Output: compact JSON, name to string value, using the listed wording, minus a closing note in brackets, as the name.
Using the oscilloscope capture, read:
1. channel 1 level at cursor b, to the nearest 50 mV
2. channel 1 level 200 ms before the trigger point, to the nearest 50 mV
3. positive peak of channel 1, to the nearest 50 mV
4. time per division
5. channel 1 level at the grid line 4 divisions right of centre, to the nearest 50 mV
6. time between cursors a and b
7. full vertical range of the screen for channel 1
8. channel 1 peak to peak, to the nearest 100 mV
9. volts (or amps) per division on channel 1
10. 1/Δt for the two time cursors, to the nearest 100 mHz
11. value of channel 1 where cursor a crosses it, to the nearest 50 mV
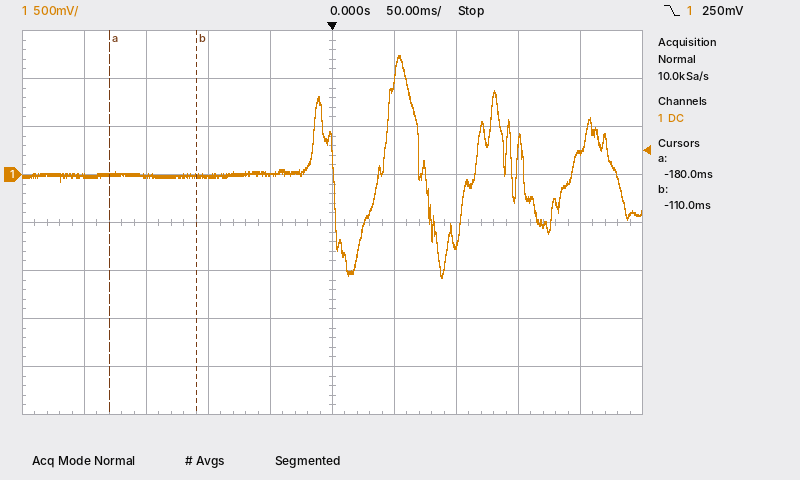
{"channel 1 level at cursor b, to the nearest 50 mV": "0 mV", "channel 1 level 200 ms before the trigger point, to the nearest 50 mV": "0 mV", "positive peak of channel 1, to the nearest 50 mV": "1.25 V", "time per division": "50 ms", "channel 1 level at the grid line 4 divisions right of centre, to the nearest 50 mV": "250 mV", "time between cursors a and b": "70 ms", "full vertical range of the screen for channel 1": "4 V", "channel 1 peak to peak, to the nearest 100 mV": "2.30 V", "volts (or amps) per division on channel 1": "500 mV", "1/Δt for the two time cursors, to the nearest 100 mHz": "14.3 Hz", "value of channel 1 where cursor a crosses it, to the nearest 50 mV": "0 mV"}
